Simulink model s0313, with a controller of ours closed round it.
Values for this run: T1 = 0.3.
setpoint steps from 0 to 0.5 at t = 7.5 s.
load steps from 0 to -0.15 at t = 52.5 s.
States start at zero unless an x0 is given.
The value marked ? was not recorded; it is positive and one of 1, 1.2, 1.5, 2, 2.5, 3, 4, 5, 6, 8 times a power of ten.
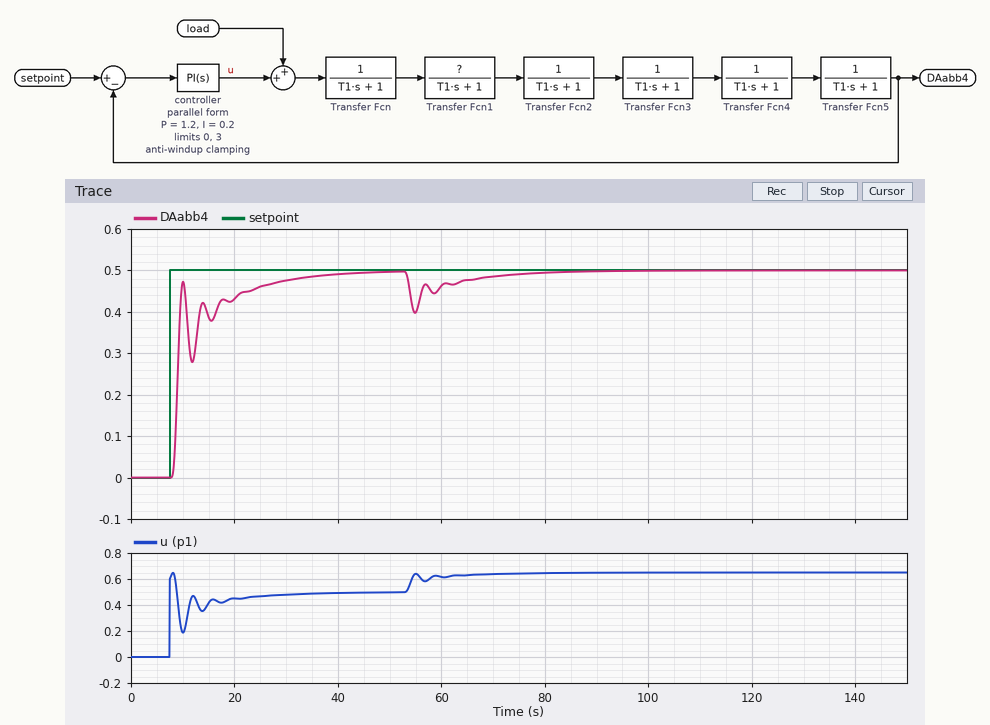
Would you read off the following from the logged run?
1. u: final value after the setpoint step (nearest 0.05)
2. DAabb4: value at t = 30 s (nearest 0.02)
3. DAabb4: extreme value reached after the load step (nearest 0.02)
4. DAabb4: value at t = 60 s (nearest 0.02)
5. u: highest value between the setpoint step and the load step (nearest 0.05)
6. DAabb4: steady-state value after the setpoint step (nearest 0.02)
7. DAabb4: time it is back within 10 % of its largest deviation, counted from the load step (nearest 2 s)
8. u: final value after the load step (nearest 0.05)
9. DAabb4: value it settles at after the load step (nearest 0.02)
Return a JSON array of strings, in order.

["0.50", "0.48", "0.40", "0.46", "0.65", "0.50", "22 s", "0.65", "0.50"]
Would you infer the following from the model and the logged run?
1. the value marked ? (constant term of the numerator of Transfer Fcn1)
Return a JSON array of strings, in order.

["1"]
